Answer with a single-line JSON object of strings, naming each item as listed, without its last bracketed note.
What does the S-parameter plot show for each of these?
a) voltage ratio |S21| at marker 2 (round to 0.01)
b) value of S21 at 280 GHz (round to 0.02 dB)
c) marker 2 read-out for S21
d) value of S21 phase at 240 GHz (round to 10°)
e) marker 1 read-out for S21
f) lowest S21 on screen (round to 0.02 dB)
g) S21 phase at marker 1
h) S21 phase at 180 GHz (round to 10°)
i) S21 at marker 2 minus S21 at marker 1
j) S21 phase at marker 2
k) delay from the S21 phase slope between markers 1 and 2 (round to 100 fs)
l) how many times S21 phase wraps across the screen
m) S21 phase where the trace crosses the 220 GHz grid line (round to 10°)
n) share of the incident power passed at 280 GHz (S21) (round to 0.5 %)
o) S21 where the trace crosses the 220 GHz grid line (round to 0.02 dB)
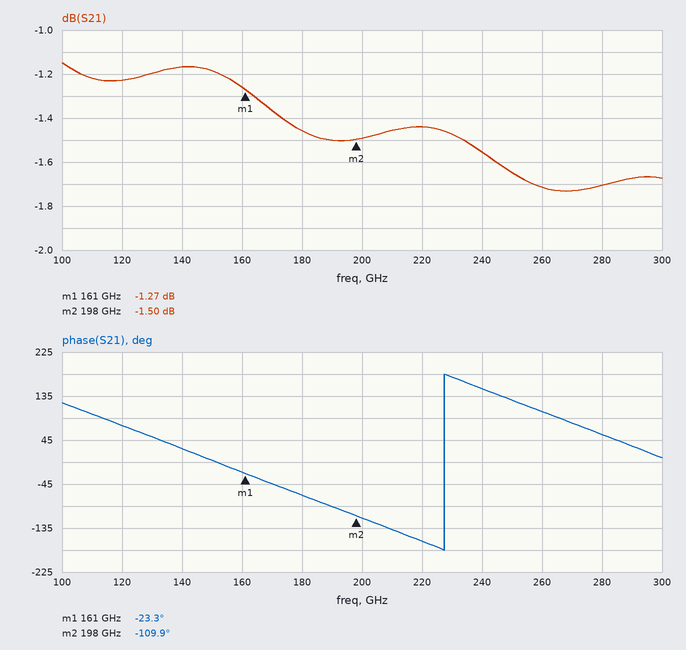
{"voltage ratio |S21| at marker 2": "0.84", "value of S21 at 280 GHz": "-1.70 dB", "marker 2 read-out for S21": "-1.50 dB", "value of S21 phase at 240 GHz": "150°", "marker 1 read-out for S21": "-1.27 dB", "lowest S21 on screen": "-1.74 dB", "S21 phase at marker 1": "-23.3°", "S21 phase at 180 GHz": "-70°", "S21 at marker 2 minus S21 at marker 1": "-0.23 dB", "S21 phase at marker 2": "-109.9°", "delay from the S21 phase slope between markers 1 and 2": "6.5 ps", "how many times S21 phase wraps across the screen": "1", "S21 phase where the trace crosses the 220 GHz grid line": "-160°", "share of the incident power passed at 280 GHz (S21)": "67.5 %", "S21 where the trace crosses the 220 GHz grid line": "-1.44 dB"}
